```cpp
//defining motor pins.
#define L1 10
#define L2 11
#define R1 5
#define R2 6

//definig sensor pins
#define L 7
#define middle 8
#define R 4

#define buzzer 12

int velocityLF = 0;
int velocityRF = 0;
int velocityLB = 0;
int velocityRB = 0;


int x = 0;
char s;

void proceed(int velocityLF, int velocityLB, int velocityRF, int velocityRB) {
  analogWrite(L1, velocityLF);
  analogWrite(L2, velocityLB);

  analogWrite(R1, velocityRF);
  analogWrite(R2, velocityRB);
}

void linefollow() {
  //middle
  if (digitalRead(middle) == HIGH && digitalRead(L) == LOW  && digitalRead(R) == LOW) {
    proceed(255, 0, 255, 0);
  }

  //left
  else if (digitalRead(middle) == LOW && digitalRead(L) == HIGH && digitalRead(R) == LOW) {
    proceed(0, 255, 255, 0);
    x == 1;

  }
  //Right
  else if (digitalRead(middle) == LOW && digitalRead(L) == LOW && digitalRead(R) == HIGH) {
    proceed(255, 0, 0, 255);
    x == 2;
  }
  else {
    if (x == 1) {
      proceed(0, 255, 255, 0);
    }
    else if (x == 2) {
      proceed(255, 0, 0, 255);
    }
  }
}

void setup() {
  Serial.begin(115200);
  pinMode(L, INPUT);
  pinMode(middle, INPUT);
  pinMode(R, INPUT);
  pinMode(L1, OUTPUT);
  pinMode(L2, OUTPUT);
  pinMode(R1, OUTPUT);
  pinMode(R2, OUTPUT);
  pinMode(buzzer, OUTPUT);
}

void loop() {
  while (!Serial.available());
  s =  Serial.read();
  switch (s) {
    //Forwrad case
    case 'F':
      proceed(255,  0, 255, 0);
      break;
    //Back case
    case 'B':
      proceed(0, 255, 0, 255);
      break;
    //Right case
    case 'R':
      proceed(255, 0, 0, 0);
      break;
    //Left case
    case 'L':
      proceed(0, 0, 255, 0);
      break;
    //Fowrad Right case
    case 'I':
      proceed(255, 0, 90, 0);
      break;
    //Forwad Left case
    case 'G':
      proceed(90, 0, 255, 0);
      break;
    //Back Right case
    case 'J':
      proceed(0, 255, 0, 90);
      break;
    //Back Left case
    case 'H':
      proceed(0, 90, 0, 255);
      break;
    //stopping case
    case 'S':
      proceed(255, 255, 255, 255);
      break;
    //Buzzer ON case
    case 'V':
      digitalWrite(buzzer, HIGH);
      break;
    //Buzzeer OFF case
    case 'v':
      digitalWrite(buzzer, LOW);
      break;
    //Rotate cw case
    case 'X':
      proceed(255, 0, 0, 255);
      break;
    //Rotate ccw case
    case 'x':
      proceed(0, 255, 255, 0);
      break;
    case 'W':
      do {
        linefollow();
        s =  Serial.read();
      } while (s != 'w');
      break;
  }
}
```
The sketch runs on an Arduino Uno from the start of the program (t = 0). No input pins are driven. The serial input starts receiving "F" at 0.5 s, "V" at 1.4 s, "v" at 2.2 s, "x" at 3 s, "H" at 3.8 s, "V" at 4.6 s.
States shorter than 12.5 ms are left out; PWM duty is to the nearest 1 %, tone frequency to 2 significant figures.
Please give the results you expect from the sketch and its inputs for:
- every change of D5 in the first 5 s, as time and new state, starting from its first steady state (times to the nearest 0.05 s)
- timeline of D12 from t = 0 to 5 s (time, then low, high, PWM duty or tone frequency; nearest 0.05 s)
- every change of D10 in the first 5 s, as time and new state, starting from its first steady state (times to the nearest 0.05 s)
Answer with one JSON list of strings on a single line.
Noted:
["0 s low; 0.5 s high; 3.8 s low", "0 s low; 1.4 s high; 2.2 s low; 4.6 s high", "0 s low; 0.5 s high; 3 s low"]
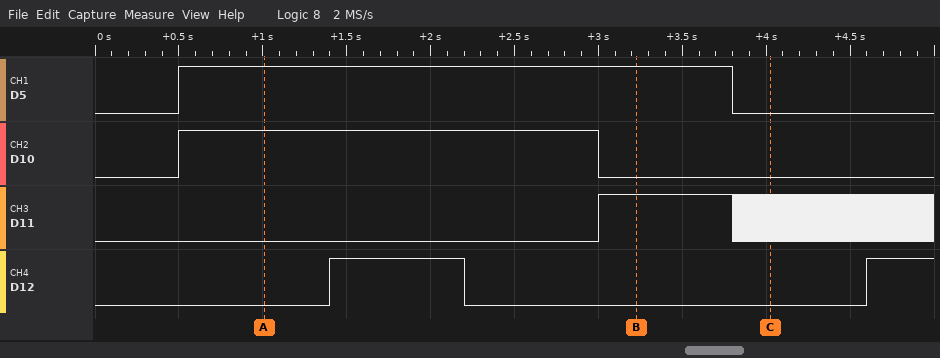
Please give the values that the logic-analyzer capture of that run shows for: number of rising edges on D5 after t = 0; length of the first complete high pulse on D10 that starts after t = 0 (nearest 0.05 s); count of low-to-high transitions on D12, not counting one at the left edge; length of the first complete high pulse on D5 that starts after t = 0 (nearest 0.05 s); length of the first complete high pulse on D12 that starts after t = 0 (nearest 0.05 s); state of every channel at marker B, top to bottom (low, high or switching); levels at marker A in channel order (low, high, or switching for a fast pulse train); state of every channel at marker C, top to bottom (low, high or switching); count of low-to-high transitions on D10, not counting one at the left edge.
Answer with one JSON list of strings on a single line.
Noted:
["1", "2.50 s", "2", "3.30 s", "0.80 s", "D5 high, D10 low, D11 high, D12 low", "D5 high, D10 high, D11 low, D12 low", "D5 low, D10 low, D11 switching, D12 low", "1"]
